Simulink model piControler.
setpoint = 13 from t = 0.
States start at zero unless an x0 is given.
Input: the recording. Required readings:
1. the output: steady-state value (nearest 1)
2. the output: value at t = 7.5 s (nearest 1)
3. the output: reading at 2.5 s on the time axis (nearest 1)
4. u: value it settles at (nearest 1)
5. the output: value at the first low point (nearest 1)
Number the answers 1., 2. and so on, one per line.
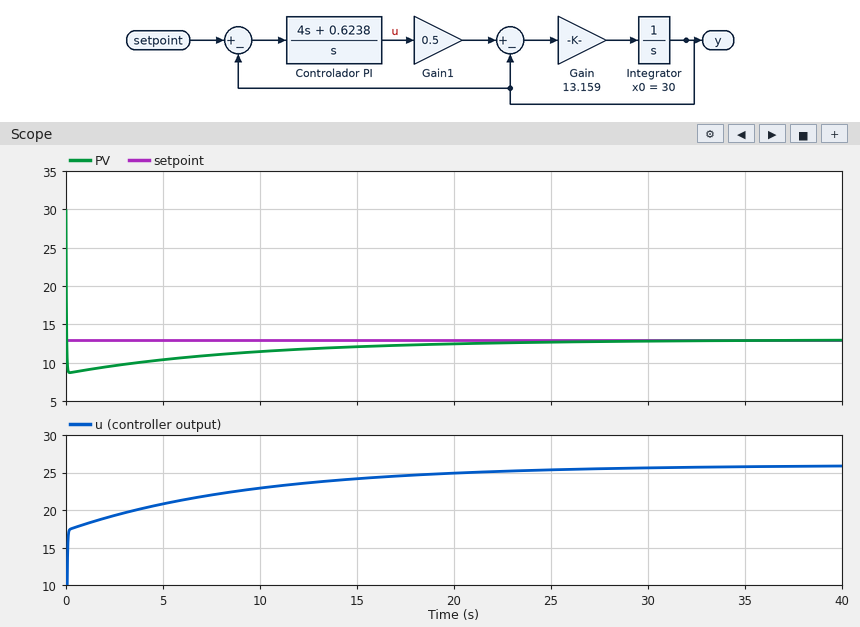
1. 13
2. 11
3. 10
4. 26
5. 9
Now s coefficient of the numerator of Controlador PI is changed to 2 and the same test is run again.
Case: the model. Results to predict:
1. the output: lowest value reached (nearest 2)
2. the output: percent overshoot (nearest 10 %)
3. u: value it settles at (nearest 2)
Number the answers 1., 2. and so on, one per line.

1. 6
2. 40 %
3. 26
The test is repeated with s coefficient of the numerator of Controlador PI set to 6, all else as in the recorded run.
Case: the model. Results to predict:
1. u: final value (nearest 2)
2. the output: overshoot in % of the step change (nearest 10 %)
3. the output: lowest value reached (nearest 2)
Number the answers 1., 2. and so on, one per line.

1. 26
2. 20 %
3. 10
